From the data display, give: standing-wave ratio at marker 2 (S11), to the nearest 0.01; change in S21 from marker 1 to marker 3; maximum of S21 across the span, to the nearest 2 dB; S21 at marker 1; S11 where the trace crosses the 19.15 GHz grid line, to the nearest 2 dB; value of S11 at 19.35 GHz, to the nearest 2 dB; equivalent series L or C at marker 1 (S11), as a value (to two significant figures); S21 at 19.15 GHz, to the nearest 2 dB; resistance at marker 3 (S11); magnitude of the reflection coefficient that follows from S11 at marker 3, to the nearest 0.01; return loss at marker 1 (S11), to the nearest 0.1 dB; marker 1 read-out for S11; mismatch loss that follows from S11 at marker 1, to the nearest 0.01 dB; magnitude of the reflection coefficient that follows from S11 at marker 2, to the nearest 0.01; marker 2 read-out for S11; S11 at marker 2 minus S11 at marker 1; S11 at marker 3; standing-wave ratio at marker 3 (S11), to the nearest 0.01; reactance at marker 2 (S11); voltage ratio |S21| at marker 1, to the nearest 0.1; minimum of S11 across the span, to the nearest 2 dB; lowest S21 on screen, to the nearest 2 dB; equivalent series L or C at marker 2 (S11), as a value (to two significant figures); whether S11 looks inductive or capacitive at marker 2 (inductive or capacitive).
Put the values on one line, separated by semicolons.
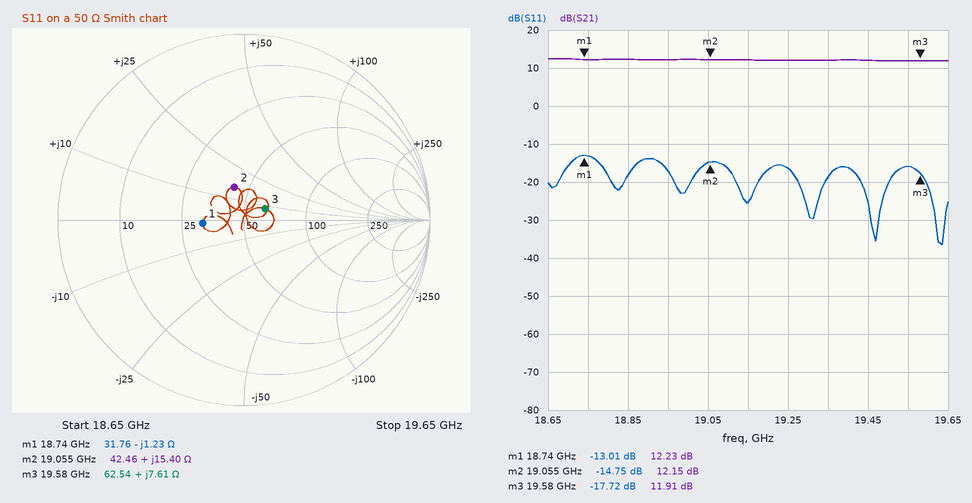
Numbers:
1.45; -0.32 dB; 12 dB; 12.23 dB; -26 dB; -18 dB; 6.9 pF; 12 dB; 62.54 Ω; 0.13; 13.0 dB; -13.01 dB; 0.22 dB; 0.18; -14.75 dB; -1.74 dB; -17.72 dB; 1.30; +15.40 Ω; 4.1; -36 dB; 12 dB; 130 pH; inductive
